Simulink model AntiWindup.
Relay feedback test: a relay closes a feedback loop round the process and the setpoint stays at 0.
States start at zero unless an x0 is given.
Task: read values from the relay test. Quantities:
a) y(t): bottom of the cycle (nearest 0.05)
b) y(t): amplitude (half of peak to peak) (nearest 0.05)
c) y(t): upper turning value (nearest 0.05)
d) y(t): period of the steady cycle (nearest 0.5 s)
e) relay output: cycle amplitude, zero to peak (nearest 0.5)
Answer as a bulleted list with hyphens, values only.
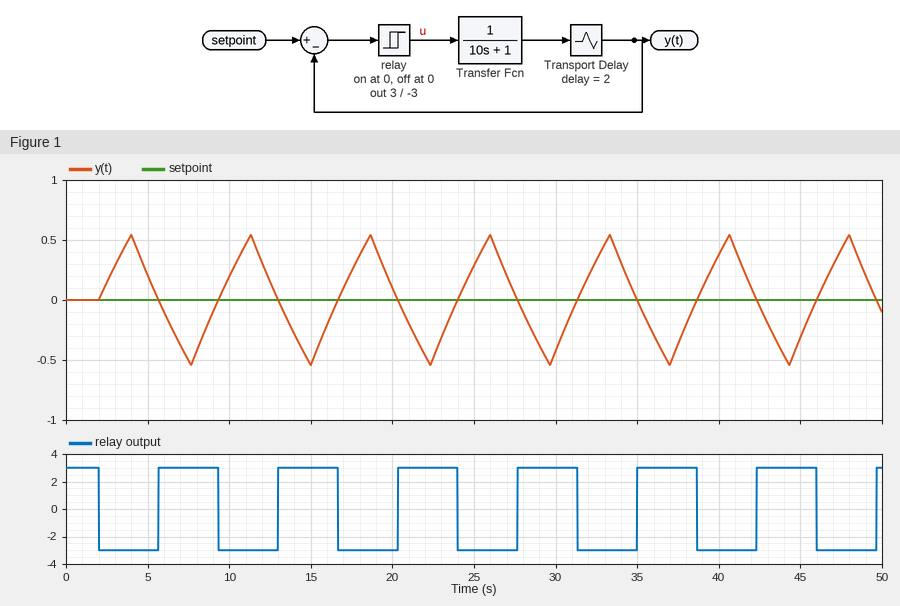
- -0.55
- 0.55
- 0.55
- 7.5 s
- 3.0
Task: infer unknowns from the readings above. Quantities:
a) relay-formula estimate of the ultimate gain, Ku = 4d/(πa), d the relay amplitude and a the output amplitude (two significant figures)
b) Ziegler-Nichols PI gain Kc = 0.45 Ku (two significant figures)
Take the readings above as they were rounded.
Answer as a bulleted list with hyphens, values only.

- 6.9
- 3.1
